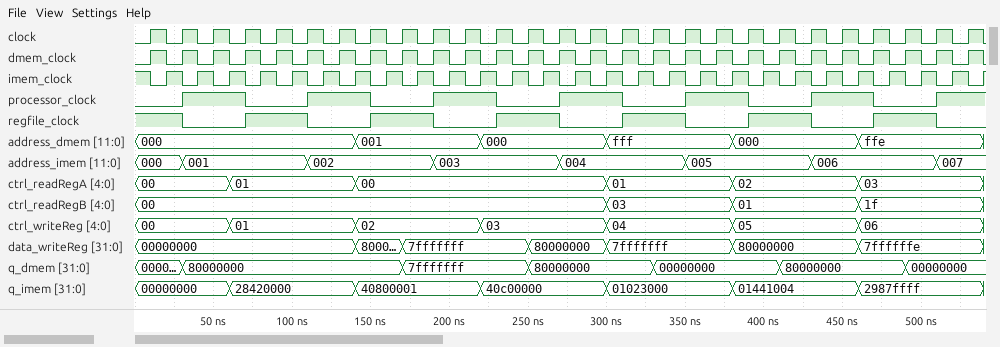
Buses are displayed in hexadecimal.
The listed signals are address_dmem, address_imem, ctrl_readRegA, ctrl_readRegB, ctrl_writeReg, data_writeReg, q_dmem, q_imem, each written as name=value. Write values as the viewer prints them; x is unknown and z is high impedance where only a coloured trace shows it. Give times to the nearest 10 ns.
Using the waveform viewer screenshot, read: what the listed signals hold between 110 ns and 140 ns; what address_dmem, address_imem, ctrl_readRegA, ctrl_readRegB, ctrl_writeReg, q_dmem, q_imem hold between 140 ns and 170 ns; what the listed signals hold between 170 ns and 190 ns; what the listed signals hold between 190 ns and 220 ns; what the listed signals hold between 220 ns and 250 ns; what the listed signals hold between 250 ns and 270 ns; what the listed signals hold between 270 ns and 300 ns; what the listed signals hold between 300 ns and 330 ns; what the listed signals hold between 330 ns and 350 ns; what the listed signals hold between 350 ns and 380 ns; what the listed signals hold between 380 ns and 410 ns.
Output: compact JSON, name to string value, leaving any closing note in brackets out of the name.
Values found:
{"what the listed signals hold between 110 ns and 140 ns": "address_dmem=000, address_imem=002, ctrl_readRegA=01, ctrl_readRegB=00, ctrl_writeReg=01, data_writeReg=00000000, q_dmem=80000000, q_imem=28420000", "what address_dmem, address_imem, ctrl_readRegA, ctrl_readRegB, ctrl_writeReg, q_dmem, q_imem hold between 140 ns and 170 ns": "address_dmem=001, address_imem=002, ctrl_readRegA=00, ctrl_readRegB=00, ctrl_writeReg=02, q_dmem=80000000, q_imem=40800001", "what the listed signals hold between 170 ns and 190 ns": "address_dmem=001, address_imem=002, ctrl_readRegA=00, ctrl_readRegB=00, ctrl_writeReg=02, data_writeReg=7fffffff, q_dmem=7fffffff, q_imem=40800001", "what the listed signals hold between 190 ns and 220 ns": "address_dmem=001, address_imem=003, ctrl_readRegA=00, ctrl_readRegB=00, ctrl_writeReg=02, data_writeReg=7fffffff, q_dmem=7fffffff, q_imem=40800001", "what the listed signals hold between 220 ns and 250 ns": "address_dmem=000, address_imem=003, ctrl_readRegA=00, ctrl_readRegB=00, ctrl_writeReg=03, data_writeReg=7fffffff, q_dmem=7fffffff, q_imem=40c00000", "what the listed signals hold between 250 ns and 270 ns": "address_dmem=000, address_imem=003, ctrl_readRegA=00, ctrl_readRegB=00, ctrl_writeReg=03, data_writeReg=80000000, q_dmem=80000000, q_imem=40c00000", "what the listed signals hold between 270 ns and 300 ns": "address_dmem=000, address_imem=004, ctrl_readRegA=00, ctrl_readRegB=00, ctrl_writeReg=03, data_writeReg=80000000, q_dmem=80000000, q_imem=40c00000", "what the listed signals hold between 300 ns and 330 ns": "address_dmem=fff, address_imem=004, ctrl_readRegA=01, ctrl_readRegB=03, ctrl_writeReg=04, data_writeReg=7fffffff, q_dmem=80000000, q_imem=01023000", "what the listed signals hold between 330 ns and 350 ns": "address_dmem=fff, address_imem=004, ctrl_readRegA=01, ctrl_readRegB=03, ctrl_writeReg=04, data_writeReg=7fffffff, q_dmem=00000000, q_imem=01023000", "what the listed signals hold between 350 ns and 380 ns": "address_dmem=fff, address_imem=005, ctrl_readRegA=01, ctrl_readRegB=03, ctrl_writeReg=04, data_writeReg=7fffffff, q_dmem=00000000, q_imem=01023000", "what the listed signals hold between 380 ns and 410 ns": "address_dmem=000, address_imem=005, ctrl_readRegA=02, ctrl_readRegB=01, ctrl_writeReg=05, data_writeReg=80000000, q_dmem=00000000, q_imem=01441004"}
